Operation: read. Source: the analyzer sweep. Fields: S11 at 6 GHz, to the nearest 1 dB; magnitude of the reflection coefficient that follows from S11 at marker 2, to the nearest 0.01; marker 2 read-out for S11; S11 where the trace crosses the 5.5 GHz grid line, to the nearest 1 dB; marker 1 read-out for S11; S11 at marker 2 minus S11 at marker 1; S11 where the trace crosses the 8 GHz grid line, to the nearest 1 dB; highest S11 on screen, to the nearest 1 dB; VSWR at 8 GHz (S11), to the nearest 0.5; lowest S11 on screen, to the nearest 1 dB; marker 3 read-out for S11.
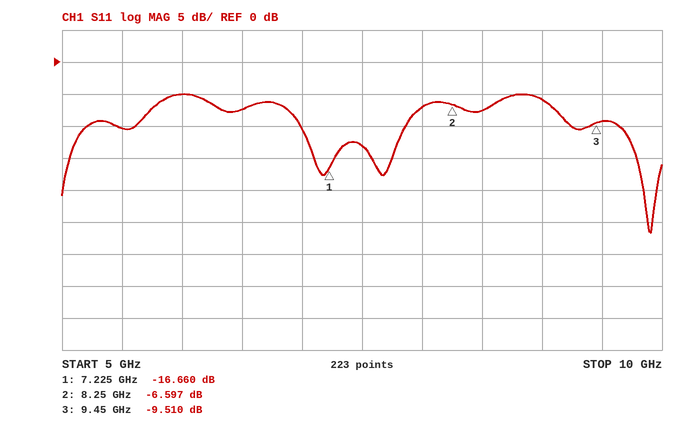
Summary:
-5 dB
0.47
-6.597 dB
-10 dB
-16.660 dB
10.063 dB
-7 dB
-5 dB
2.5
-27 dB
-9.510 dB
